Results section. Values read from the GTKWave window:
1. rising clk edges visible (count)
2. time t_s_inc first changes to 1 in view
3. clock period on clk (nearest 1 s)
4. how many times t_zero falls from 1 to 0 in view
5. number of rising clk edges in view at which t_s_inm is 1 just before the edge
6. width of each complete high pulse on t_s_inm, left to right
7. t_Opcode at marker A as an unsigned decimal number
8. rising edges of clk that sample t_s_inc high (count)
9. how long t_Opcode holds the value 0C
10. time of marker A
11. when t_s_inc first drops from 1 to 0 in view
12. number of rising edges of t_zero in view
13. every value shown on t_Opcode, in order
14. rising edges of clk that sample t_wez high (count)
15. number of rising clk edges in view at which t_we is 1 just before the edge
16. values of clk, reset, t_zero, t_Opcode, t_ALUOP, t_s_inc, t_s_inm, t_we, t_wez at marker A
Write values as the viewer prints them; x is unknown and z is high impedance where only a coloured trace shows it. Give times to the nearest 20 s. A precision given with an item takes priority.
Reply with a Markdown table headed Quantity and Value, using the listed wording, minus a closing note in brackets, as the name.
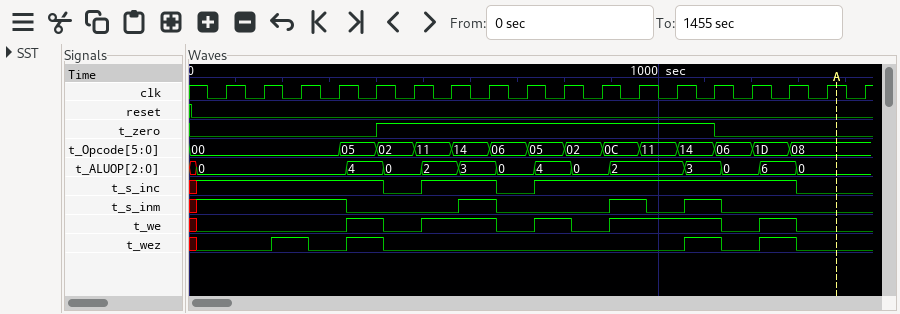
| Quantity | Value |
|---|---|
| rising clk edges visible | 18 |
| time t_s_inc first changes to 1 in view | 20 s |
| clock period on clk | 80 s |
| how many times t_zero falls from 1 to 0 in view | 1 |
| number of rising clk edges in view at which t_s_inm is 1 just before the edge | 7 |
| width of each complete high pulse on t_s_inm, left to right | 80 s, 80 s, 80 s |
| t_Opcode at marker A as an unsigned decimal number | 8 |
| rising edges of clk that sample t_s_inc high | 14 |
| how long t_Opcode holds the value 0C | 80 s |
| time of marker A | 1380 s |
| when t_s_inc first drops from 1 to 0 in view | 420 s |
| number of rising edges of t_zero in view | 1 |
| every value shown on t_Opcode, in order | 00, 05, 02, 11, 14, 06, 05, 02, 0C, 11, 14, 06, 1D, 08 |
| rising edges of clk that sample t_wez high | 4 |
| number of rising clk edges in view at which t_we is 1 just before the edge | 8 |
| values of clk, reset, t_zero, t_Opcode, t_ALUOP, t_s_inc, t_s_inm, t_we, t_wez at marker A | clk=1, reset=0, t_zero=0, t_Opcode=08, t_ALUOP=0, t_s_inc=0, t_s_inm=0, t_we=0, t_wez=0 |
